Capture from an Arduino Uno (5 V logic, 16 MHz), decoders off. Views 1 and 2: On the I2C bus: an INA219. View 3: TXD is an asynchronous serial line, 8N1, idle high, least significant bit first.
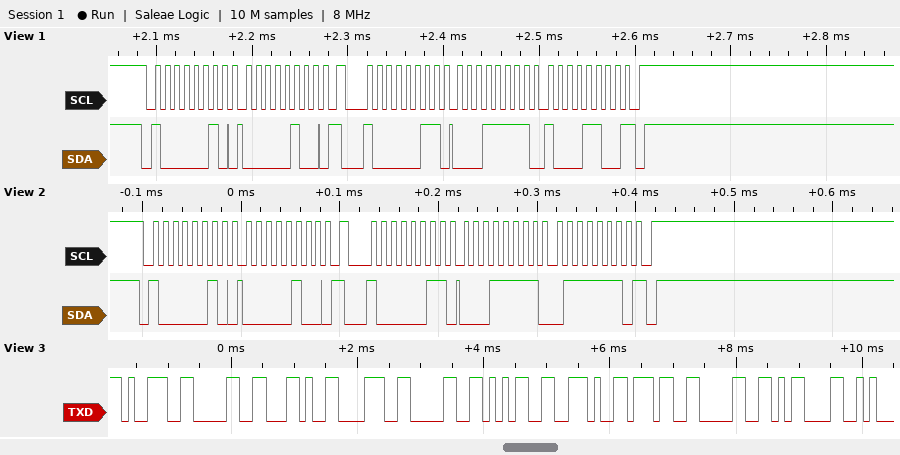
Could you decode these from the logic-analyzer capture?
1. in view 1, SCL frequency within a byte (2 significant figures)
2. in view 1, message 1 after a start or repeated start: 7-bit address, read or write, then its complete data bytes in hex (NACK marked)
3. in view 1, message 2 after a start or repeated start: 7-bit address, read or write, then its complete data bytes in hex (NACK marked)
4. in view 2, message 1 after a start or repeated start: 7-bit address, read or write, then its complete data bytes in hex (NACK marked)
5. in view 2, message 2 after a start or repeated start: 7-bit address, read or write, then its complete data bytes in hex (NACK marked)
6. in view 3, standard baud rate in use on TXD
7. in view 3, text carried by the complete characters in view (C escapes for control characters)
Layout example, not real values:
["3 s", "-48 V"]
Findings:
["100 kHz", "0x41 write: 04", "0x41 read: 1F 8C NACK", "0x41 write: 04", "0x41 read: 1F 7E NACK", "9600 baud", "\"90,805.70\\r\""]
